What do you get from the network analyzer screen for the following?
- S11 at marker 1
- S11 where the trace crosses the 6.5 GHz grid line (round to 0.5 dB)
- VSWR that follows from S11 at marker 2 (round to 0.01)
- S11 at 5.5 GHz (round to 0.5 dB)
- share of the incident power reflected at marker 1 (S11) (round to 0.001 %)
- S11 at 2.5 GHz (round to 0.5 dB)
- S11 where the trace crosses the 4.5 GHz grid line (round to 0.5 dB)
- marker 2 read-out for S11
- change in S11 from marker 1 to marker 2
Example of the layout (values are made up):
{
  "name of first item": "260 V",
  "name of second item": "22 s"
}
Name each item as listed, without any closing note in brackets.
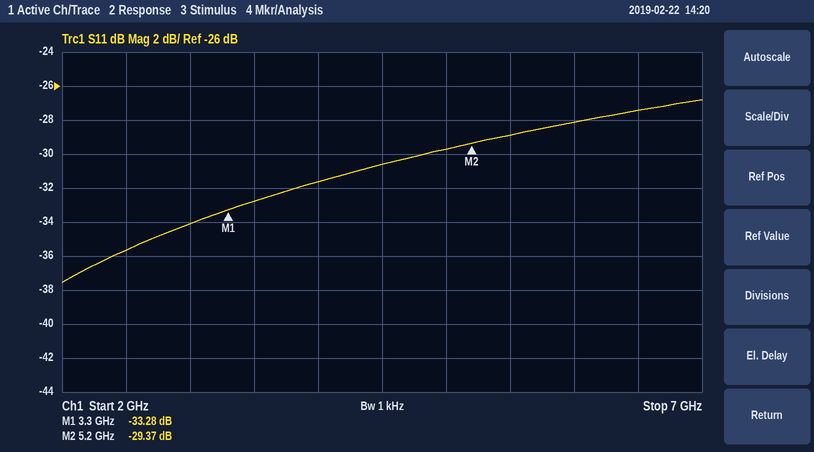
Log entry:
{
  "S11 at marker 1": "-33.28 dB",
  "S11 where the trace crosses the 6.5 GHz grid line": "-27.5 dB",
  "VSWR that follows from S11 at marker 2": "1.07",
  "S11 at 5.5 GHz": "-29.0 dB",
  "share of the incident power reflected at marker 1 (S11)": "0.047 %",
  "S11 at 2.5 GHz": "-35.5 dB",
  "S11 where the trace crosses the 4.5 GHz grid line": "-30.5 dB",
  "marker 2 read-out for S11": "-29.37 dB",
  "change in S11 from marker 1 to marker 2": "3.91 dB"
}
